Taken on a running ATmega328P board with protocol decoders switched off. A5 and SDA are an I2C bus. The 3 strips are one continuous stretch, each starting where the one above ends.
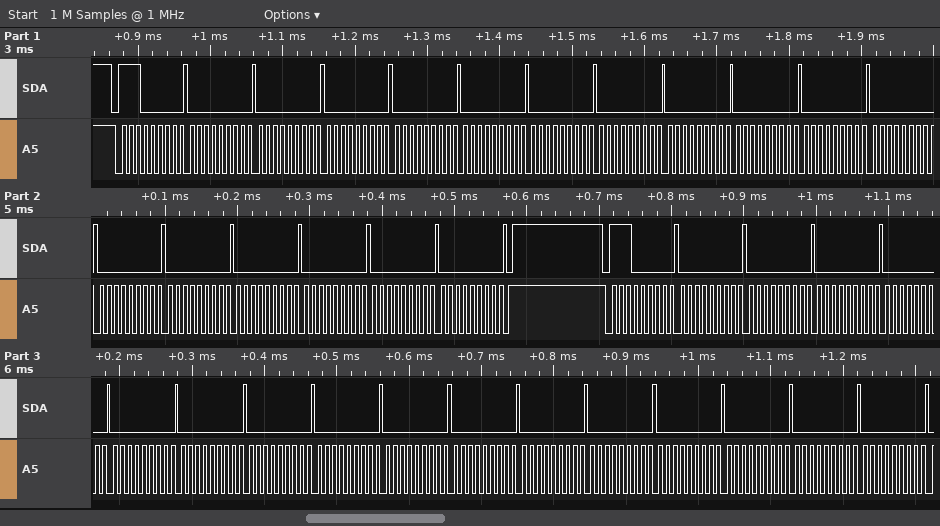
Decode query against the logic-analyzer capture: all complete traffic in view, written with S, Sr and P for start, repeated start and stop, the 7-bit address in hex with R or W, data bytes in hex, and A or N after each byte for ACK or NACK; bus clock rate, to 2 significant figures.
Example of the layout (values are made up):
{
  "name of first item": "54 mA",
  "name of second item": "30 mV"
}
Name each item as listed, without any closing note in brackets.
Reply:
{
  "all complete traffic in view, written with S, Sr and P for start, repeated start and stop, the 7-bit address in hex with R or W, data bytes in hex, and A or N after each byte for ACK or NACK": "S 70W A 00 A 00 A 00 A 00 A 00 A 00 A 00 A 00 A 00 A 00 A 00 A 00 A 00 A 00 A 00 A 00 A 00 A P S 70W A 00 A 00 A 00 A 00 A 00 A 00 A 00 A 00 A 00 A 00 A 00 A 00 A 00 A 00 A 00 A 00 A",
  "bus clock rate, to 2 significant figures": "100 kHz"
}
